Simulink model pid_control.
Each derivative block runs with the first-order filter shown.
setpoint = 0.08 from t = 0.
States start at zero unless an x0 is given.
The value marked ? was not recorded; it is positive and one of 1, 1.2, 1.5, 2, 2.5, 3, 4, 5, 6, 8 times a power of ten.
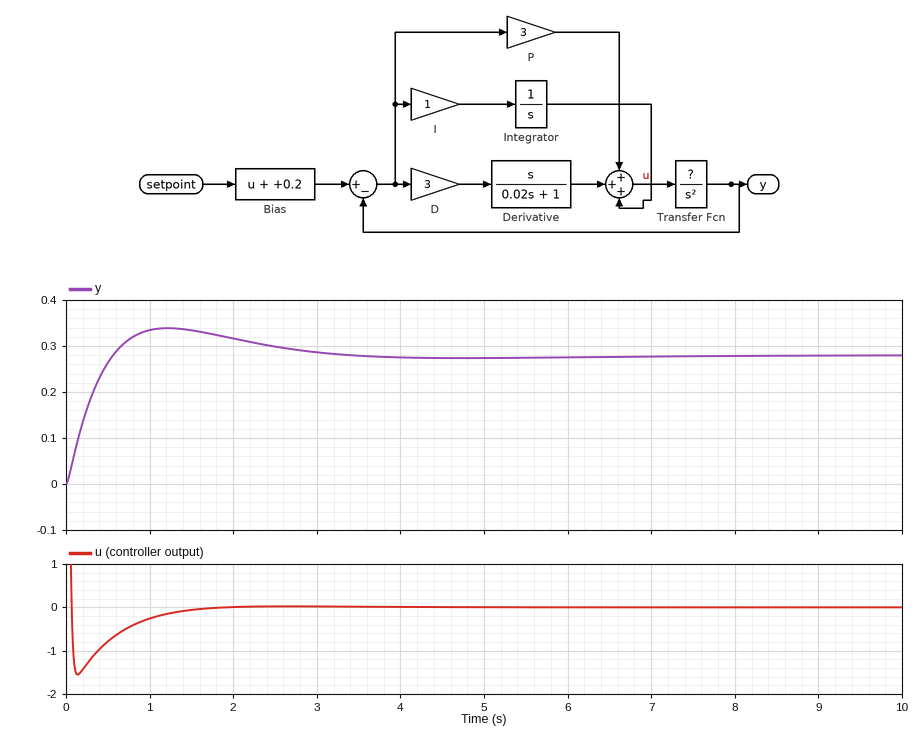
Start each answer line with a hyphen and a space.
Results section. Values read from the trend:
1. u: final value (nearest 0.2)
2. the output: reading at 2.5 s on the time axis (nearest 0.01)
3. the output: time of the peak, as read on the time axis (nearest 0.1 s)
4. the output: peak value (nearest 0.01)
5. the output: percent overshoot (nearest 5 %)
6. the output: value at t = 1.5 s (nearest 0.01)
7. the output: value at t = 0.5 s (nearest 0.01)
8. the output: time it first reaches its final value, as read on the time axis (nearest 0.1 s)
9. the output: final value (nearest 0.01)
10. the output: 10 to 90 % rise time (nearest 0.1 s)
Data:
- 0.0
- 0.30
- 1.2 s
- 0.34
- 20 %
- 0.33
- 0.26
- 0.6 s
- 0.28
- 0.4 s
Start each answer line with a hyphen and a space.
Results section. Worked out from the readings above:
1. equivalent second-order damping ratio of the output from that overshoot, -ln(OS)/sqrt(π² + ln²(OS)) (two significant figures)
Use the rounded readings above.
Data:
- 0.46
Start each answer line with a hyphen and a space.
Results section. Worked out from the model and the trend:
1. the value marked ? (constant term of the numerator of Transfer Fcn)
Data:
- 1
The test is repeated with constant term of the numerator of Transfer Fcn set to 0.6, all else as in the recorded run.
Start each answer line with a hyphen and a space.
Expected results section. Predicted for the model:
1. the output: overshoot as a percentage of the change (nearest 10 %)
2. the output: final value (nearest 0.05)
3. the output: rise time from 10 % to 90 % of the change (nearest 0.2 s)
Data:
- 30 %
- 0.30
- 0.6 s
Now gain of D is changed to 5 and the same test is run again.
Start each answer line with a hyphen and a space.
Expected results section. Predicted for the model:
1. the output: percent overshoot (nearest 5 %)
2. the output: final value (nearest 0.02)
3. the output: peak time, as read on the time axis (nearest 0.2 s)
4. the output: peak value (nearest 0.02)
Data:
- 10 %
- 0.28
- 1.0 s
- 0.30
